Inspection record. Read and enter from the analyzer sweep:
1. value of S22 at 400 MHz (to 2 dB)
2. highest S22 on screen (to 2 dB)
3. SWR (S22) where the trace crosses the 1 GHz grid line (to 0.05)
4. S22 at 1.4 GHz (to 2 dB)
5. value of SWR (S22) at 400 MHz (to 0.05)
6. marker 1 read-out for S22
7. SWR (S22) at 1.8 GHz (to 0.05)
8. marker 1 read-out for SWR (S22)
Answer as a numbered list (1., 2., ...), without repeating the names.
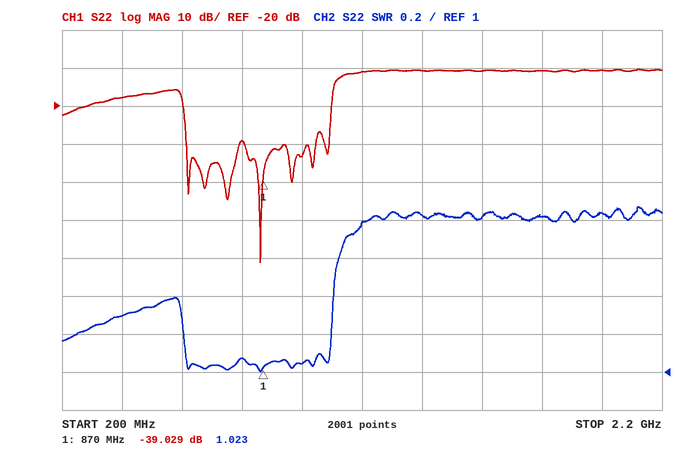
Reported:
1. -18 dB
2. -10 dB
3. 1.05
4. -10 dB
5. 1.30
6. -39.029 dB
7. 1.80
8. 1.023
